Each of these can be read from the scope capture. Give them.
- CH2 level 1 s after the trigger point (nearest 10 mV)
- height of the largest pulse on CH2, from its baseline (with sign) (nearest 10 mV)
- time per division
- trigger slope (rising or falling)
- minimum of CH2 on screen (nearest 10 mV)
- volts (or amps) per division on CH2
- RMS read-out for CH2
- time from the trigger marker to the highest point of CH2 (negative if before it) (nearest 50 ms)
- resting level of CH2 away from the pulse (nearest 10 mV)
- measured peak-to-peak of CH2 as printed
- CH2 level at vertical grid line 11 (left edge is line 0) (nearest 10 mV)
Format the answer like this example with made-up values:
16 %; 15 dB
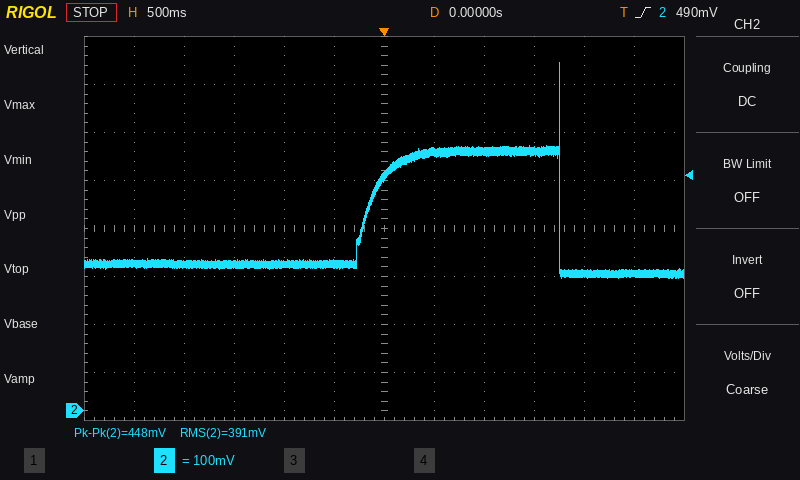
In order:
540 mV; +420 mV; 500 ms; rising; 280 mV; 100 mV; 391 mV; +1.75 s; 310 mV; 448 mV; 290 mV
